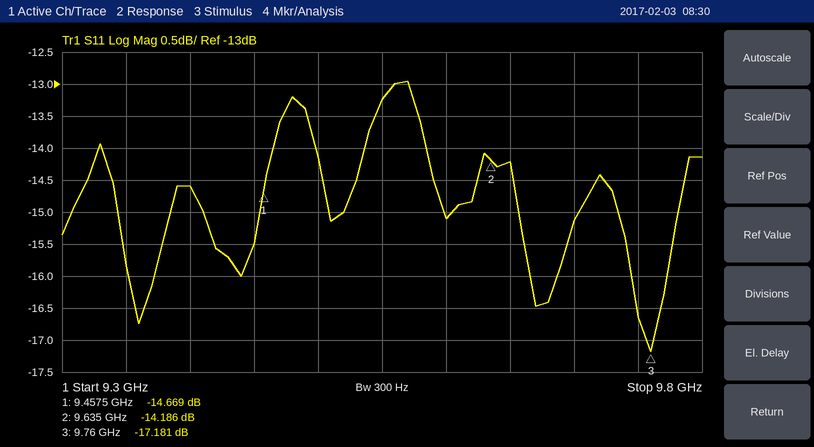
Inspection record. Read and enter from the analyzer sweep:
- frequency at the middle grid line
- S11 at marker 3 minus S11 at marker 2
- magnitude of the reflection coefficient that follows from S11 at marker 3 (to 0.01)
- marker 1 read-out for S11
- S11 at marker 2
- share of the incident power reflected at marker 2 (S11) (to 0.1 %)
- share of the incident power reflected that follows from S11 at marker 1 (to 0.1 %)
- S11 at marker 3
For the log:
9.55 GHz
-2.995 dB
0.14
-14.669 dB
-14.186 dB
3.8 %
3.4 %
-17.181 dB
